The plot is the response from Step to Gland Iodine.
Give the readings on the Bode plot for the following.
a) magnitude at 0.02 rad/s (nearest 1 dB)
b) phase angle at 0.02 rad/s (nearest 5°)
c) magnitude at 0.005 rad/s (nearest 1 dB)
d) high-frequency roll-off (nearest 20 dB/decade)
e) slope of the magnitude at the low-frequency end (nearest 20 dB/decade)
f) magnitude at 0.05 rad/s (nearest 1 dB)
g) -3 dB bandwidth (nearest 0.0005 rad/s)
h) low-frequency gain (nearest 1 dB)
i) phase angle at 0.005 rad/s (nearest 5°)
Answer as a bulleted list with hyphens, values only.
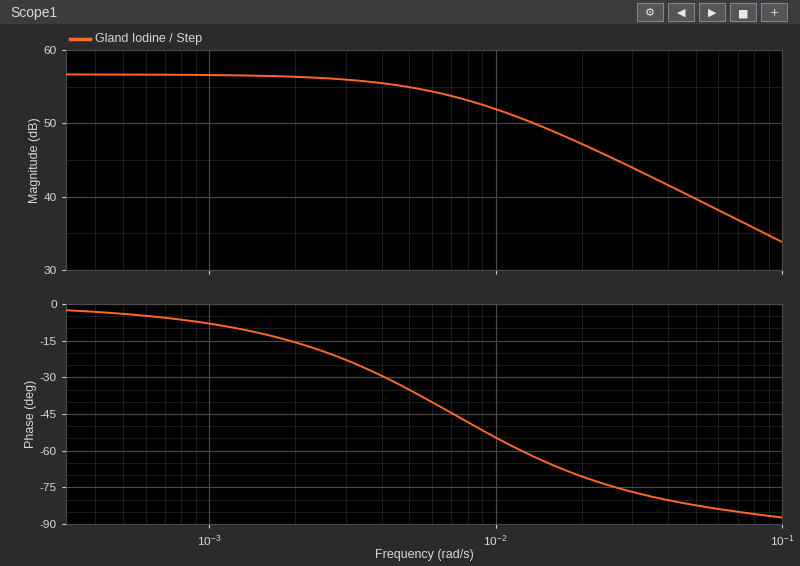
- 47 dB
- -70°
- 55 dB
- -20 dB/decade
- 0 dB/decade
- 40 dB
- 0.0070 rad/s
- 57 dB
- -35°
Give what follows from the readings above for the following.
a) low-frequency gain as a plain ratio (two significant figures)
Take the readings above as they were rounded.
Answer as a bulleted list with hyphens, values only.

- 710
